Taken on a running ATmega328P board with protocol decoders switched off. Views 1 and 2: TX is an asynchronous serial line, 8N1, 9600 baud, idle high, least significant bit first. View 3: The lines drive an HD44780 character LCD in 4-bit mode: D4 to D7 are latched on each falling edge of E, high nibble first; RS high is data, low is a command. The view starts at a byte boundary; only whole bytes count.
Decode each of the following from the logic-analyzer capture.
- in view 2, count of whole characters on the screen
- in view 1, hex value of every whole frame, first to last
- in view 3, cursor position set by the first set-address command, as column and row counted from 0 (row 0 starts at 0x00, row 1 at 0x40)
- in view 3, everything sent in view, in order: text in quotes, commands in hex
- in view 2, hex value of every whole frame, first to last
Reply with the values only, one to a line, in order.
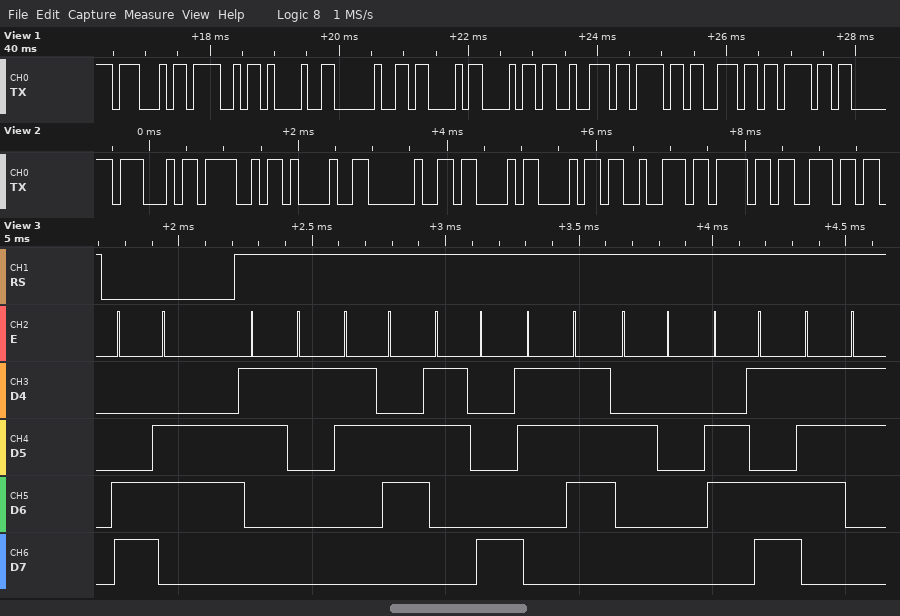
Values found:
9
47 4F 21 20 43 68 72 6F 6E 6F
column 6, row 1
0xC6 "1687 ms"
0x47 0x4F 0x21 0x20 0x43 0x68 0x72 0x6F 0x6E
